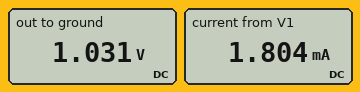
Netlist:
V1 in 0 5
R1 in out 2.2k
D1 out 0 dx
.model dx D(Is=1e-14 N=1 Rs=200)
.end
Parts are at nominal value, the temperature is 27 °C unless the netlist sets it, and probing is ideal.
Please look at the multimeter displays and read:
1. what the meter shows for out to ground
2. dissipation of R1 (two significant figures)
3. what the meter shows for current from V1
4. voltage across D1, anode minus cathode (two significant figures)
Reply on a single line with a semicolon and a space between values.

1.031 V; 7.2 mW; 1.804 mA; 1.0 V
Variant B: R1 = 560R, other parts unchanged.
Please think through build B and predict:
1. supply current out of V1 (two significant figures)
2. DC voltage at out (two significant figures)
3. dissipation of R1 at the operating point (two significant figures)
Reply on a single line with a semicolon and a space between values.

5.7 mA; 1.8 V; 18 mW
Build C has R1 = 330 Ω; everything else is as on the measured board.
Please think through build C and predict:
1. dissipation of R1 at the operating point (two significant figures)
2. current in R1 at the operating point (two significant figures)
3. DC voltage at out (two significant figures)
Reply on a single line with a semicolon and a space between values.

22 mW; 8.1 mA; 2.3 V
